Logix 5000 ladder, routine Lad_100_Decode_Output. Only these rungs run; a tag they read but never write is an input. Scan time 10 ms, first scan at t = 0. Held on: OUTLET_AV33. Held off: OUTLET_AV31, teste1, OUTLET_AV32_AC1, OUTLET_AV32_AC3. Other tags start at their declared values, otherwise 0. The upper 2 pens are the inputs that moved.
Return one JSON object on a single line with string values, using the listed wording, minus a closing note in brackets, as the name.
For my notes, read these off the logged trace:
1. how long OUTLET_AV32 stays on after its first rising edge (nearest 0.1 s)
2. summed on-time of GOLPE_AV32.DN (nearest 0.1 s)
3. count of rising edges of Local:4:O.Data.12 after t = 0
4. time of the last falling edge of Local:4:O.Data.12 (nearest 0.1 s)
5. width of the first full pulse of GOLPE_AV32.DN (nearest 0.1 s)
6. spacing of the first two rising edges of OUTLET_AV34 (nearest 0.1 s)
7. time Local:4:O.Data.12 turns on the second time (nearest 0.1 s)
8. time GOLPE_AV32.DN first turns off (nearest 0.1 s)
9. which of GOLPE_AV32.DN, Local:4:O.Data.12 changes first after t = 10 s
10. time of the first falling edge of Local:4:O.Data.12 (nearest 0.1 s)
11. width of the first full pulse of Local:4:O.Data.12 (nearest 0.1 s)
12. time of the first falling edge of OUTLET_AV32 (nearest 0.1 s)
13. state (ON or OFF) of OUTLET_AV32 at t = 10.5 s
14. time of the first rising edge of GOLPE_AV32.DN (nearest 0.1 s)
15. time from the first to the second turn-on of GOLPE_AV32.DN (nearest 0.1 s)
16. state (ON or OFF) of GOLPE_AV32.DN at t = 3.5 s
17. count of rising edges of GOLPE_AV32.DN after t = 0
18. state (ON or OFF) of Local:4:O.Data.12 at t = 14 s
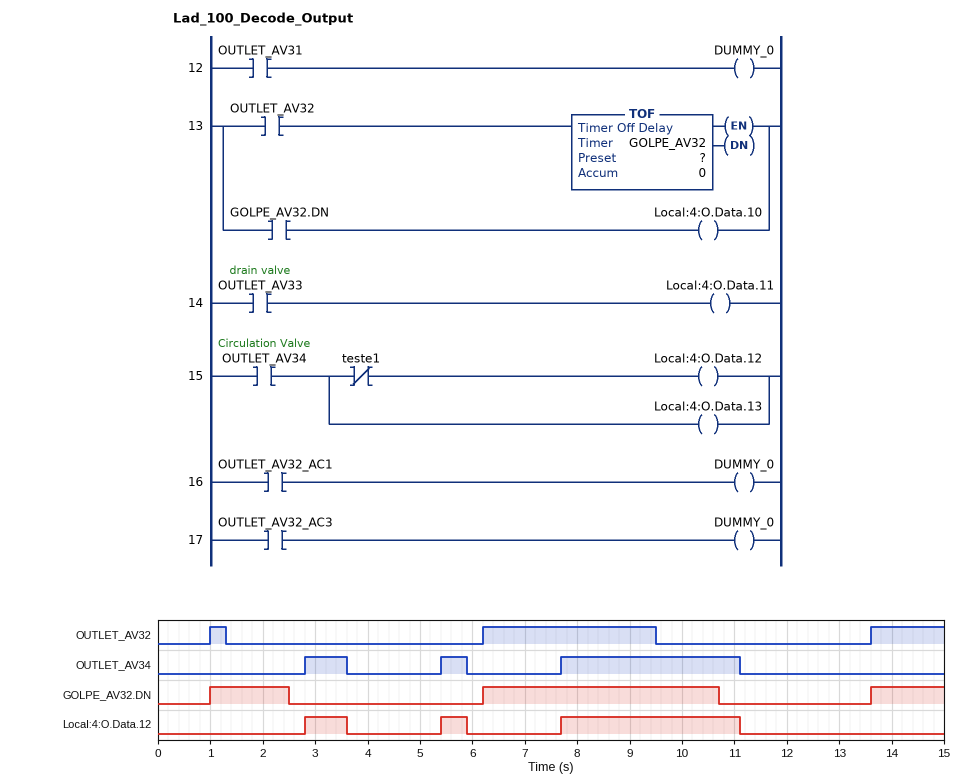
{"how long OUTLET_AV32 stays on after its first rising edge": "0.3 s", "summed on-time of GOLPE_AV32.DN": "7.4 s", "count of rising edges of Local:4:O.Data.12 after t = 0": "3", "time of the last falling edge of Local:4:O.Data.12": "11.1 s", "width of the first full pulse of GOLPE_AV32.DN": "1.5 s", "spacing of the first two rising edges of OUTLET_AV34": "2.6 s", "time Local:4:O.Data.12 turns on the second time": "5.4 s", "time GOLPE_AV32.DN first turns off": "2.5 s", "which of GOLPE_AV32.DN, Local:4:O.Data.12 changes first after t = 10 s": "GOLPE_AV32.DN", "time of the first falling edge of Local:4:O.Data.12": "3.6 s", "width of the first full pulse of Local:4:O.Data.12": "0.8 s", "time of the first falling edge of OUTLET_AV32": "1.3 s", "state (ON or OFF) of OUTLET_AV32 at t = 10.5 s": "OFF", "time of the first rising edge of GOLPE_AV32.DN": "1.0 s", "time from the first to the second turn-on of GOLPE_AV32.DN": "5.2 s", "state (ON or OFF) of GOLPE_AV32.DN at t = 3.5 s": "OFF", "count of rising edges of GOLPE_AV32.DN after t = 0": "3", "state (ON or OFF) of Local:4:O.Data.12 at t = 14 s": "OFF"}
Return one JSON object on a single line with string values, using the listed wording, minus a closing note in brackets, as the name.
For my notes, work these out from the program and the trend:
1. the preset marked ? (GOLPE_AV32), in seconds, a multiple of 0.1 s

{"the preset marked ? (GOLPE_AV32), in seconds, a multiple of 0.1 s": "1.2 s"}
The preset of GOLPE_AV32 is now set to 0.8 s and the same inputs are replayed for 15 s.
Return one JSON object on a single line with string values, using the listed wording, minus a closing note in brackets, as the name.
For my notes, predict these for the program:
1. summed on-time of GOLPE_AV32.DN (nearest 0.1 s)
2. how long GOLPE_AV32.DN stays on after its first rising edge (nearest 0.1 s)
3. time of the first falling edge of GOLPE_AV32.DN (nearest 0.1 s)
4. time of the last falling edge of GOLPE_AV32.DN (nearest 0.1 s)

{"summed on-time of GOLPE_AV32.DN": "6.6 s", "how long GOLPE_AV32.DN stays on after its first rising edge": "1.1 s", "time of the first falling edge of GOLPE_AV32.DN": "2.1 s", "time of the last falling edge of GOLPE_AV32.DN": "10.3 s"}
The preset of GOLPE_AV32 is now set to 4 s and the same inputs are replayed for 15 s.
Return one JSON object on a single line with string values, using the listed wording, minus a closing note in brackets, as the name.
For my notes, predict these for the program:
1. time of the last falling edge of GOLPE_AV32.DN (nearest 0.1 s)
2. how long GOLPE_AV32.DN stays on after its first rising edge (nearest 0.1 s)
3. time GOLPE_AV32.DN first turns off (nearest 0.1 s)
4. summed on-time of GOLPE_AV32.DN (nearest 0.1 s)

{"time of the last falling edge of GOLPE_AV32.DN": "13.5 s", "how long GOLPE_AV32.DN stays on after its first rising edge": "4.3 s", "time GOLPE_AV32.DN first turns off": "5.3 s", "summed on-time of GOLPE_AV32.DN": "13.0 s"}
